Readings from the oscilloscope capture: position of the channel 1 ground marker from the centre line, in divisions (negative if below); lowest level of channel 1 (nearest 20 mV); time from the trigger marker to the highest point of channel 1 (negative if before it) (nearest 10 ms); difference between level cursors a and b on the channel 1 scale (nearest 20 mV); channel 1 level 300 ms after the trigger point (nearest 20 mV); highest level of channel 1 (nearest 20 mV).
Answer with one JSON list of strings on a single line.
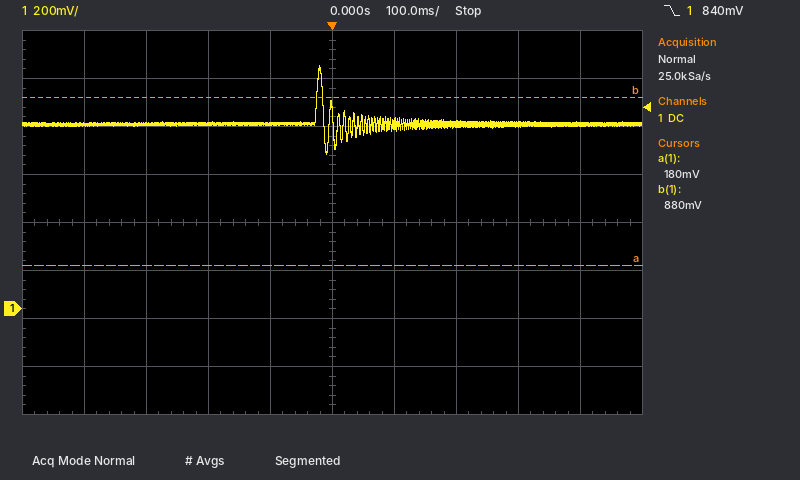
["-1.8 div", "640 mV", "-20 ms", "700 mV", "760 mV", "1.02 V"]
